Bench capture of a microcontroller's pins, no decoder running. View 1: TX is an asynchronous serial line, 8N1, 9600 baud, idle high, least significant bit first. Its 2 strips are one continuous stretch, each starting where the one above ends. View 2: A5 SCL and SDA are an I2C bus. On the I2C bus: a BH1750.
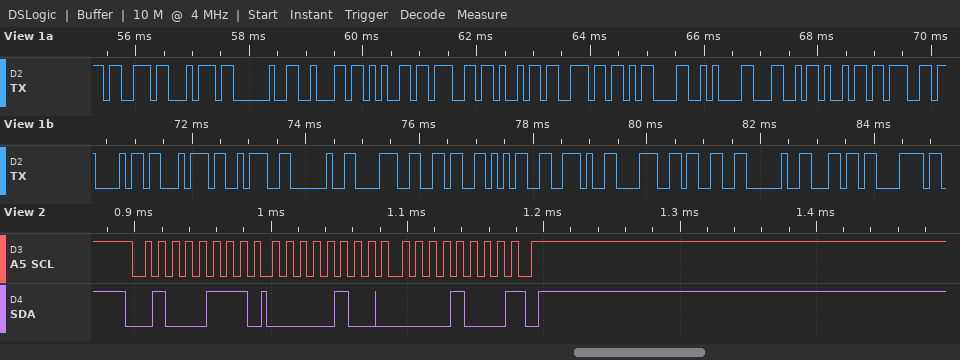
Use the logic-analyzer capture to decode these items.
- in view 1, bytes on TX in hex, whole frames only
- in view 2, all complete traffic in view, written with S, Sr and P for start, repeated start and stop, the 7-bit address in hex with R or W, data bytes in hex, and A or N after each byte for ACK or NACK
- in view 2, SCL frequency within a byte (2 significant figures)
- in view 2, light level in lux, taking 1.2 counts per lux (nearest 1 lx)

73 74 20 62 65 67 69 6E 0D 0A 4C 69 67 68 74 3A 20 38 36 35 2E 38 33 20 6C 78
S 23R A 04 A 08 N P
100 kHz
860 lx
